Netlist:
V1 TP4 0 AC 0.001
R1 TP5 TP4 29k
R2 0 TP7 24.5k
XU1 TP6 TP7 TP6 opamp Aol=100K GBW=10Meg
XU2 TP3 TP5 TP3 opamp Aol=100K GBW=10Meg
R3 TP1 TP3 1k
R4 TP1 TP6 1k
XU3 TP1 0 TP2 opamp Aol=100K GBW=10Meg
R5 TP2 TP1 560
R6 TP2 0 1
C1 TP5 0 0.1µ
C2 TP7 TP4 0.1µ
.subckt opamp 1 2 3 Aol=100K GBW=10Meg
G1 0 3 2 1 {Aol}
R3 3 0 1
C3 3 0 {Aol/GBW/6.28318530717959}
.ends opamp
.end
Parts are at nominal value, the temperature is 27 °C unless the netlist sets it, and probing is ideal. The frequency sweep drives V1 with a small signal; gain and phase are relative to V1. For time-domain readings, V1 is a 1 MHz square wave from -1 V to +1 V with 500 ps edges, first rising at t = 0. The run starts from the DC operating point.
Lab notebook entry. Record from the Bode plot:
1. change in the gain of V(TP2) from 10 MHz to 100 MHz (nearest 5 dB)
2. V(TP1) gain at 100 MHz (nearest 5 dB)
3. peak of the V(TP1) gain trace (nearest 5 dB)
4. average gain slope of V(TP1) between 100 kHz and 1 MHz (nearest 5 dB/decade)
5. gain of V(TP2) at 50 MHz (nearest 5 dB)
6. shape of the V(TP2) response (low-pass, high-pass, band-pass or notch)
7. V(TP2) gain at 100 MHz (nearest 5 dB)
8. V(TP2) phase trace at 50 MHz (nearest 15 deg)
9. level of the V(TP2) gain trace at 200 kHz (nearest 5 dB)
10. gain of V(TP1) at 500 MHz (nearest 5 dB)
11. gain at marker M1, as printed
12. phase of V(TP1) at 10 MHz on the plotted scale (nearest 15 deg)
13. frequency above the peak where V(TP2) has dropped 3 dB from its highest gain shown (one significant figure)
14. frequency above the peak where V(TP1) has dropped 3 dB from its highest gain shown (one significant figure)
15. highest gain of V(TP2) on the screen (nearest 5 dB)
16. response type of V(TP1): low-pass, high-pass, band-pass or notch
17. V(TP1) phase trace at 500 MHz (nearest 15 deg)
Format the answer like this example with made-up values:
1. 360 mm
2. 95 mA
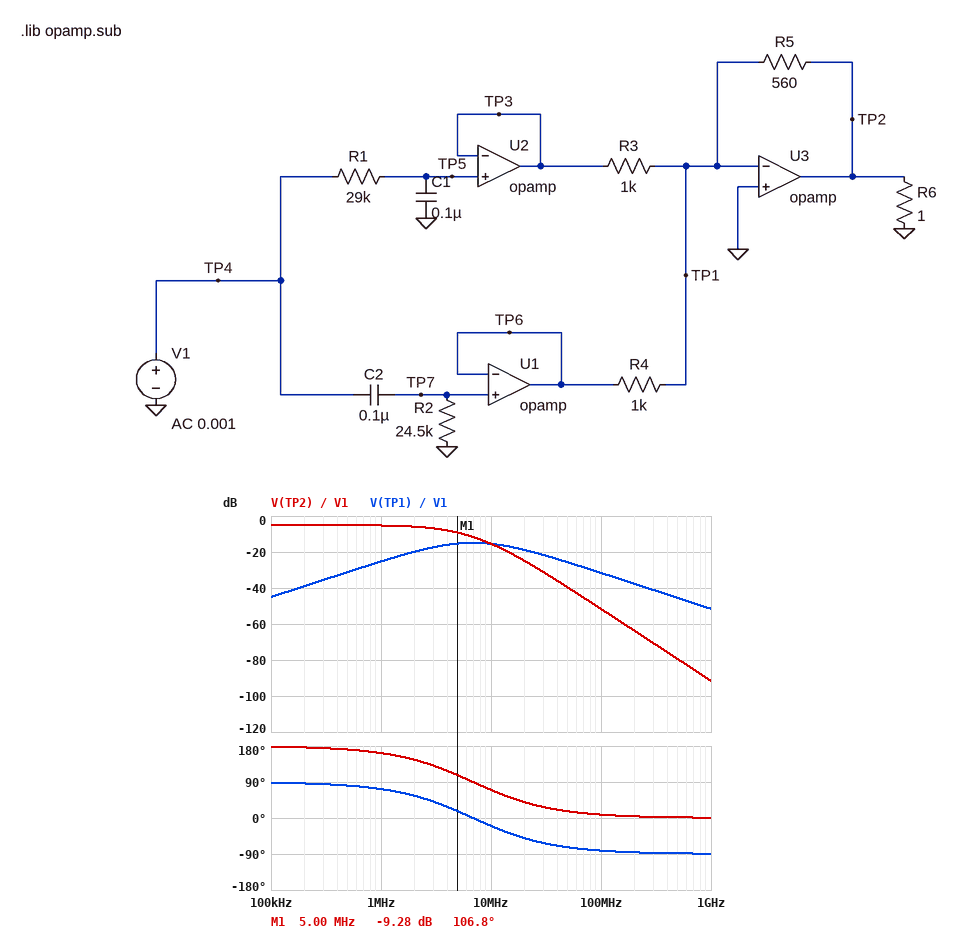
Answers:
1. -35 dB
2. -30 dB
3. -15 dB
4. 20 dB/decade
5. -40 dB
6. low-pass
7. -50 dB
8. 15 deg
9. -5 dB
10. -45 dB
11. -9.28 dB
12. -15 deg
13. 4 MHz
14. 20 MHz
15. -5 dB
16. band-pass
17. -90 deg
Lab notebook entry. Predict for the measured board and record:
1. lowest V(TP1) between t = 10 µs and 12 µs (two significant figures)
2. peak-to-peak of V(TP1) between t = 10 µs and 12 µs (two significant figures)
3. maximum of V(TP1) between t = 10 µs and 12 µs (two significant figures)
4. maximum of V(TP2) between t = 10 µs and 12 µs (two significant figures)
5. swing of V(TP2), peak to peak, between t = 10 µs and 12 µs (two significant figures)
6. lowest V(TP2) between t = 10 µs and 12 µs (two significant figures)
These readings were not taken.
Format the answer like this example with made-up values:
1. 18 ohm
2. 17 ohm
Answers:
1. -270 mV
2. 540 mV
3. 270 mV
4. 560 mV
5. 1.1 V
6. -560 mV
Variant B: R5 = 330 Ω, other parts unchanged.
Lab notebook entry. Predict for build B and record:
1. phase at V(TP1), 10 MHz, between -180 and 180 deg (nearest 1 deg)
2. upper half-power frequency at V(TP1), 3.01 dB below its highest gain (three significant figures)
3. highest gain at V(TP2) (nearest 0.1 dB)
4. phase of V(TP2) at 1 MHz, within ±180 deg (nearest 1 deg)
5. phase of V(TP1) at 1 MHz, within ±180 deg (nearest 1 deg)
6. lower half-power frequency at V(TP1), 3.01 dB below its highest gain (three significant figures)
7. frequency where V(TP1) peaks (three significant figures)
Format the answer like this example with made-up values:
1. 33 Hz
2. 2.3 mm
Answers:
1. -14 deg
2. 19.2 MHz
3. -9.6 dB
4. 165 deg
5. 75 deg
6. 3.14 MHz
7. 7.76 MHz
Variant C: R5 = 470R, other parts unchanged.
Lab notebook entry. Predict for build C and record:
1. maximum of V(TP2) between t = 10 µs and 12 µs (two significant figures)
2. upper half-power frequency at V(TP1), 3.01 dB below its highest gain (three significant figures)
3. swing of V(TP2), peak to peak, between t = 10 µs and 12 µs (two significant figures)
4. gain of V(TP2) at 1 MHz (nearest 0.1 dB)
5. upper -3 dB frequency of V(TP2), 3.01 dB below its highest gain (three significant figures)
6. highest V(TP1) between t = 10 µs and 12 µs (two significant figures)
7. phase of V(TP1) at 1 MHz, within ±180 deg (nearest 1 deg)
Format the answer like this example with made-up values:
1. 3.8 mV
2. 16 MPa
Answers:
1. 470 mV
2. 18.0 MHz
3. 940 mV
4. -6.8 dB
5. 4.28 MHz
6. 240 mV
7. 73 deg
